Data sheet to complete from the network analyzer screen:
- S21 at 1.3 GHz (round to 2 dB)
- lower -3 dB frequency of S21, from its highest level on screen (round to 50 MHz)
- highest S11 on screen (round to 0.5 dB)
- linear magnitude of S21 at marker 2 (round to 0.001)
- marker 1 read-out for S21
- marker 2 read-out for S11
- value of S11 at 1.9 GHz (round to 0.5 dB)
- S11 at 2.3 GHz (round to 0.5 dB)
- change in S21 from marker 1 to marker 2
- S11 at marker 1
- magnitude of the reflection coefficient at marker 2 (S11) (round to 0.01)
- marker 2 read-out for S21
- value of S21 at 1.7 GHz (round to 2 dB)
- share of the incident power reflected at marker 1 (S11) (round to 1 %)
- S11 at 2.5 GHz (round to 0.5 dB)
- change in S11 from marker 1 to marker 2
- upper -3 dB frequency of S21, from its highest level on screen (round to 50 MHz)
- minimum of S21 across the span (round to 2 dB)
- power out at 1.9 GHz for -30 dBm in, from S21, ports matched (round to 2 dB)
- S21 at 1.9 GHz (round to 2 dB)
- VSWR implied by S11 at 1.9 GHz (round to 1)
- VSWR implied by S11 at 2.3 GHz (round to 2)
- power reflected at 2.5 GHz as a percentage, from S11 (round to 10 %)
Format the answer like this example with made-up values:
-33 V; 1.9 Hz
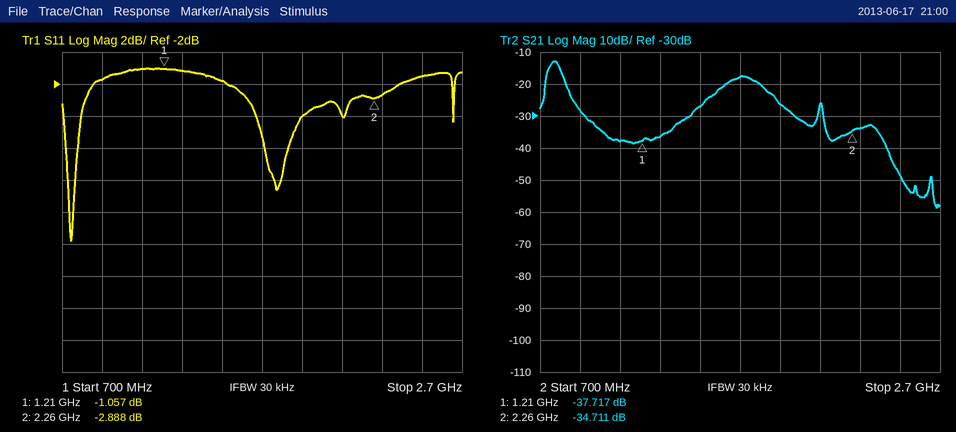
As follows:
-36 dB; 750 MHz; -1.0 dB; 0.018; -37.717 dB; -2.888 dB; -4.0 dB; -2.5 dB; 3.006 dB; -1.057 dB; 0.72; -34.711 dB; -18 dB; 78 %; -1.5 dB; -1.831 dB; 800 MHz; -58 dB; -56 dBm; -26 dB; 4; 6; 70 %
